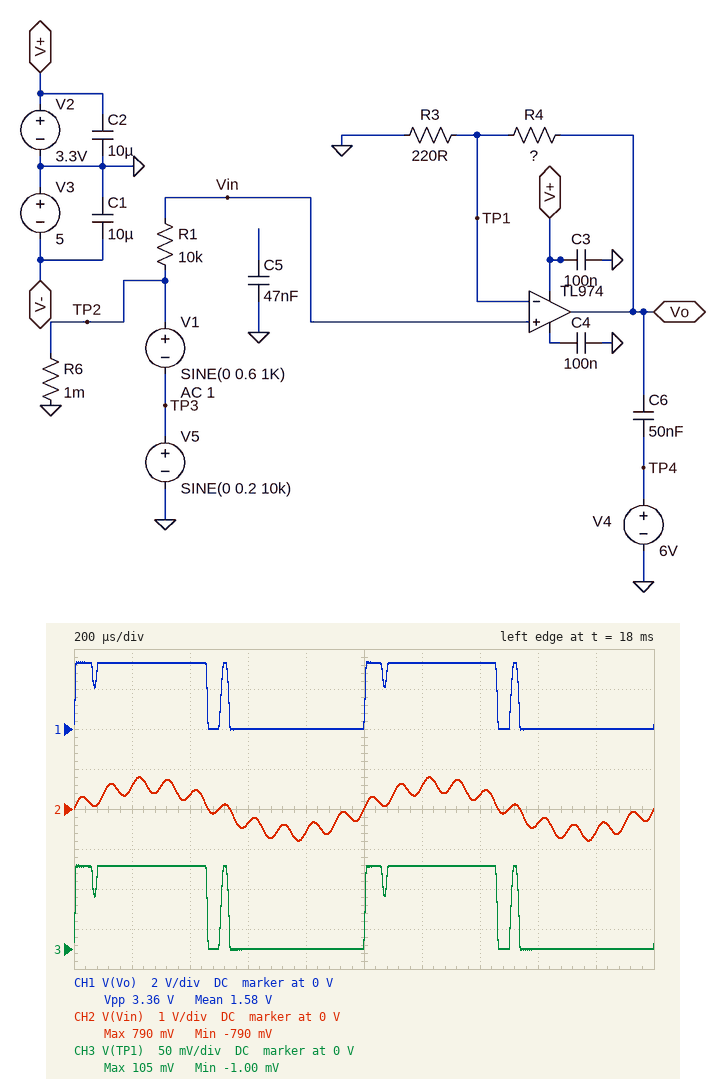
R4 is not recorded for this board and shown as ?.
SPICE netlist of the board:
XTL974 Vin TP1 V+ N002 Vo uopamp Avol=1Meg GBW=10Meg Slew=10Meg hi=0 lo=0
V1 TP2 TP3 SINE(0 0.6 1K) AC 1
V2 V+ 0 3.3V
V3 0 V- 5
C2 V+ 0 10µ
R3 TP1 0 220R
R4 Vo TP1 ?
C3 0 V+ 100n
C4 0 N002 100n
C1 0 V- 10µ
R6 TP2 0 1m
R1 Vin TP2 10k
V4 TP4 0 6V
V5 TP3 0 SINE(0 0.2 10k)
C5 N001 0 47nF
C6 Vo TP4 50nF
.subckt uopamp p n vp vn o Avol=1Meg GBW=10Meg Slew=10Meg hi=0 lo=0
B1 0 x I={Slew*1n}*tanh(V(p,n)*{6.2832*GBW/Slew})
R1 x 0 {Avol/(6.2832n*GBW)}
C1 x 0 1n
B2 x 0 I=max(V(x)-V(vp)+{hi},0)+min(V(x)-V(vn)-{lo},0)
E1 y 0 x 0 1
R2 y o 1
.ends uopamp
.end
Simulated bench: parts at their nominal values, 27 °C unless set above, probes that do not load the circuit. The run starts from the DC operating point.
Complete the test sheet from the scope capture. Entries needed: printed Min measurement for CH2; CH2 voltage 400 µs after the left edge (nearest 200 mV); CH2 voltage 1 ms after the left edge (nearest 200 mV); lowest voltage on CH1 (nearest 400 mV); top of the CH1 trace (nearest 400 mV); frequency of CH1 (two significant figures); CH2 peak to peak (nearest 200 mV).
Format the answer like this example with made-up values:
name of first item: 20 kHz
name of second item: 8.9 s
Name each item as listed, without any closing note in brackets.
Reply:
printed Min measurement for CH2: -790 mV
CH2 voltage 400 µs after the left edge: 400 mV
CH2 voltage 1 ms after the left edge: 0 V
lowest voltage on CH1: 0 V
top of the CH1 trace: 3.2 V
frequency of CH1: 2.0 kHz
CH2 peak to peak: 1.6 V
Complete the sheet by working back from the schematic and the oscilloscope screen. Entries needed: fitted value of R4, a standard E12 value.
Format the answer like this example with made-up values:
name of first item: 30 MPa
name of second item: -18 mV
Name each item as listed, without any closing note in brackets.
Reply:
fitted value of R4, a standard E12 value: 6.8 kΩ
